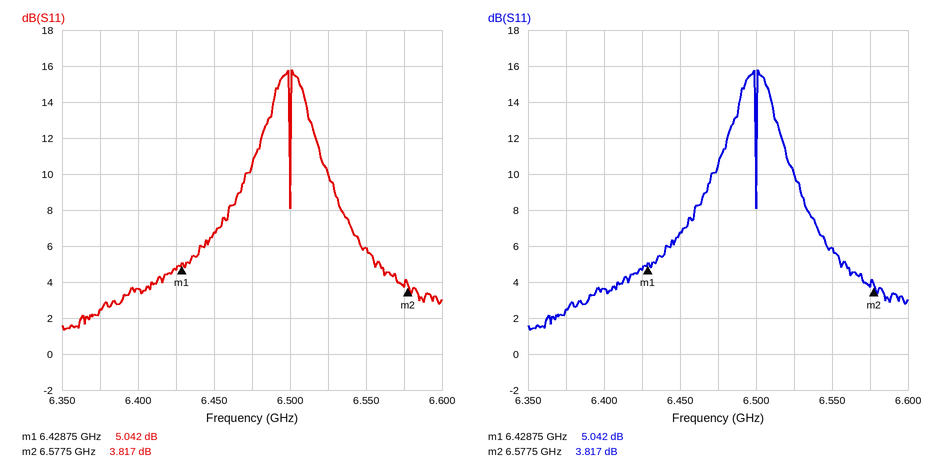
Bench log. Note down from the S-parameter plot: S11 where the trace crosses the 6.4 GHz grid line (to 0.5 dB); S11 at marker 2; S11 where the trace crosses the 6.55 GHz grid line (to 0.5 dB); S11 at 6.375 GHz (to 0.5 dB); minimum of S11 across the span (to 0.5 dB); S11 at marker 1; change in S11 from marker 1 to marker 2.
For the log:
3.5 dB
3.817 dB
6.0 dB
2.5 dB
1.5 dB
5.042 dB
-1.225 dB
